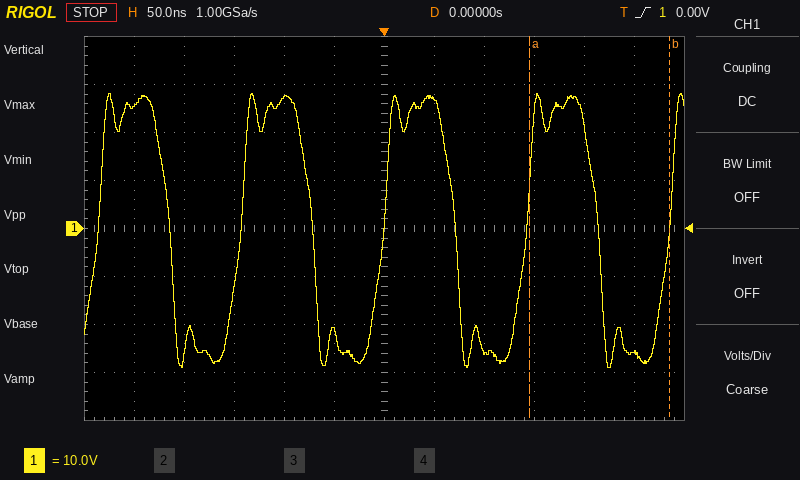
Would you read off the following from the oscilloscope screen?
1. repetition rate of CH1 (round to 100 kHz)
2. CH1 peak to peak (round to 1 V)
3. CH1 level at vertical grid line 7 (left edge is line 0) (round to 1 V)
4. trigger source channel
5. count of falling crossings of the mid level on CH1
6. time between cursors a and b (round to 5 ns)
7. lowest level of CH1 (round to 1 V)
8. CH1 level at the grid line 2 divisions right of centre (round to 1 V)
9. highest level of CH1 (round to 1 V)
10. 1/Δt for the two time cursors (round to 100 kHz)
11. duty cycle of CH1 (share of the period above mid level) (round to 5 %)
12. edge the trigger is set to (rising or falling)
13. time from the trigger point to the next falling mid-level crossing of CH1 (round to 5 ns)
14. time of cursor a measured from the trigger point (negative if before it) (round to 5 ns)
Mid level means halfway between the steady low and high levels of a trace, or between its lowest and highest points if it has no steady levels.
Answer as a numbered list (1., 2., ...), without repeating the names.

1. 7.0 MHz
2. 57 V
3. 27 V
4. CH1
5. 4
6. 140 ns
7. -29 V
8. -25 V
9. 28 V
10. 7.1 MHz
11. 50 %
12. rising
13. 70 ns
14. +145 ns
